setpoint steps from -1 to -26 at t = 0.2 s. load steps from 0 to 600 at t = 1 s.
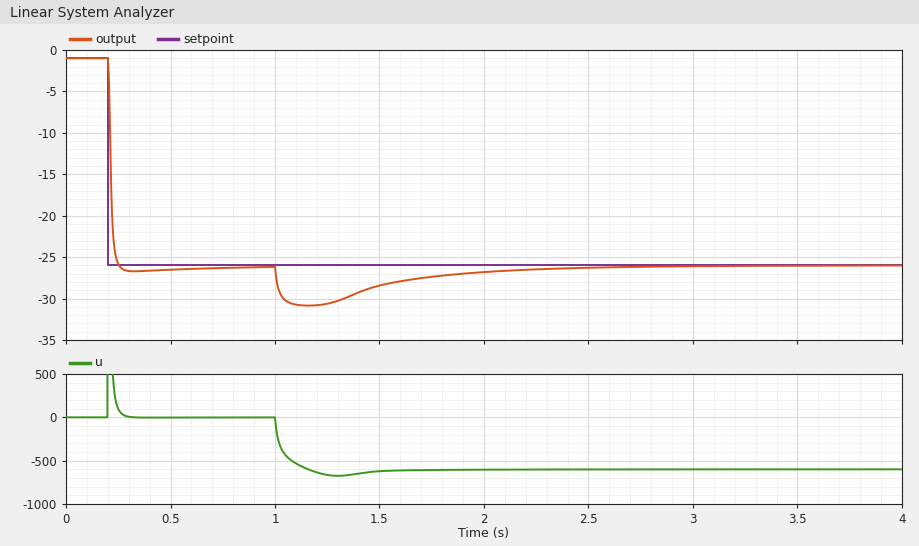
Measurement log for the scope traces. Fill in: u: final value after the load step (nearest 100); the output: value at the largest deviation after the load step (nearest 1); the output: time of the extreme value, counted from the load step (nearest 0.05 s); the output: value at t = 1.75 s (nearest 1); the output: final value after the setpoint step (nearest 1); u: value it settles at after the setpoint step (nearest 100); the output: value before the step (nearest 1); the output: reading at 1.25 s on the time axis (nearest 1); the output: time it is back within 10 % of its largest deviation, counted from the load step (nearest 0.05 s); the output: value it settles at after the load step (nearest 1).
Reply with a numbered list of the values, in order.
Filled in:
1. -600
2. -31
3. 0.15 s
4. -27
5. -26
6. 0
7. -1
8. -31
9. 1.25 s
10. -26
